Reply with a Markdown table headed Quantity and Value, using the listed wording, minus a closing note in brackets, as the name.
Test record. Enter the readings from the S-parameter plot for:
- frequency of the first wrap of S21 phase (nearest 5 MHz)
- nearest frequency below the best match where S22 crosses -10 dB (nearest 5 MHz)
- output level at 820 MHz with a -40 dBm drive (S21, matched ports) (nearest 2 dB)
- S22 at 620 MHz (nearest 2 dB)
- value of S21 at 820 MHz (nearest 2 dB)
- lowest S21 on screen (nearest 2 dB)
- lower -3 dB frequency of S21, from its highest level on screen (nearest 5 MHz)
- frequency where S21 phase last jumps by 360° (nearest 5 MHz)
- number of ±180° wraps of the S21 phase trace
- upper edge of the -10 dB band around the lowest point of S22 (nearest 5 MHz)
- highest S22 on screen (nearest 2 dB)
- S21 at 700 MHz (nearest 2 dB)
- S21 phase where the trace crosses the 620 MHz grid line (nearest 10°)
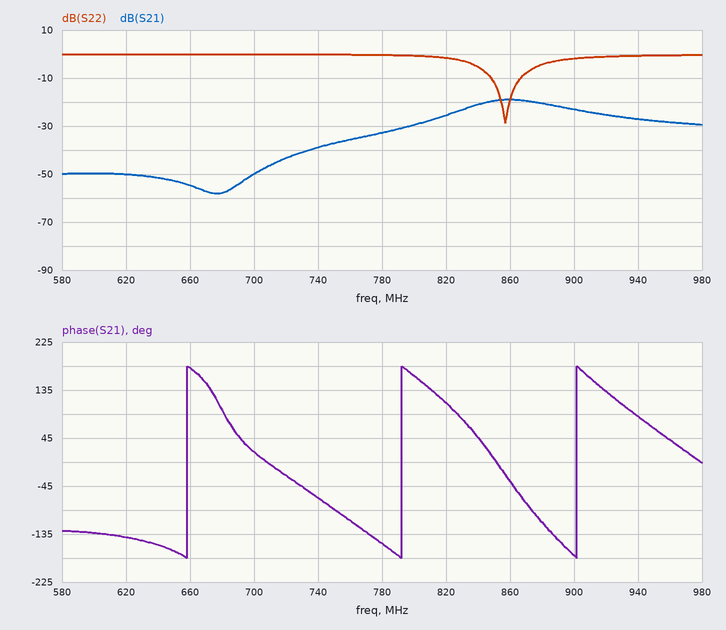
| Quantity | Value |
|---|---|
| frequency of the first wrap of S21 phase | 660 MHz |
| nearest frequency below the best match where S22 crosses -10 dB | 850 MHz |
| output level at 820 MHz with a -40 dBm drive (S21, matched ports) | -66 dBm |
| S22 at 620 MHz | 0 dB |
| value of S21 at 820 MHz | -26 dB |
| lowest S21 on screen | -58 dB |
| lower -3 dB frequency of S21, from its highest level on screen | 835 MHz |
| frequency where S21 phase last jumps by 360° | 900 MHz |
| number of ±180° wraps of the S21 phase trace | 3 |
| upper edge of the -10 dB band around the lowest point of S22 | 865 MHz |
| highest S22 on screen | 0 dB |
| S21 at 700 MHz | -50 dB |
| S21 phase where the trace crosses the 620 MHz grid line | -140° |
